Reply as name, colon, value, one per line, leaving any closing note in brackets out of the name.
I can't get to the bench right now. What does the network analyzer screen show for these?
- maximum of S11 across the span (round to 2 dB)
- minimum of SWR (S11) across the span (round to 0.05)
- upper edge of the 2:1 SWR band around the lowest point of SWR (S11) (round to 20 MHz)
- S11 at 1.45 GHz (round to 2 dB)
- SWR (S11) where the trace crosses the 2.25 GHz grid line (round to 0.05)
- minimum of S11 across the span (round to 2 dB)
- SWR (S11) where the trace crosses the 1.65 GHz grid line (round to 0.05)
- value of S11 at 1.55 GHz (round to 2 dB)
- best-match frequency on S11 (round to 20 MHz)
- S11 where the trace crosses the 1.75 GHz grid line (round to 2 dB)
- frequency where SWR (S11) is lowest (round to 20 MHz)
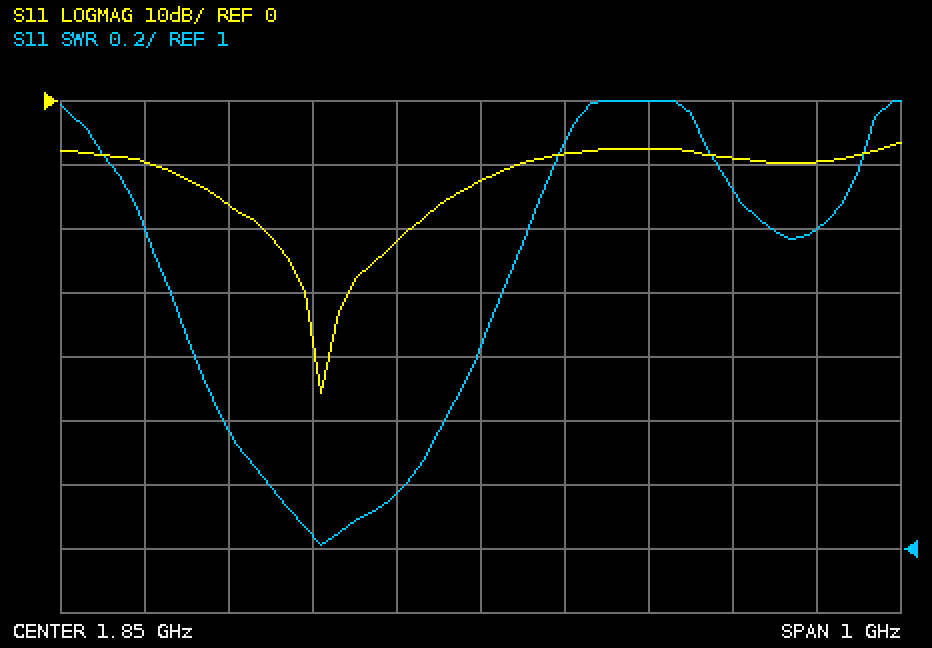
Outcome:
maximum of S11 across the span: -6 dB
minimum of SWR (S11) across the span: 1.00
upper edge of the 2:1 SWR band around the lowest point of SWR (S11): 1.90 GHz
S11 at 1.45 GHz: -10 dB
SWR (S11) where the trace crosses the 2.25 GHz grid line: 2.00
minimum of S11 across the span: -46 dB
SWR (S11) where the trace crosses the 1.65 GHz grid line: 1.05
value of S11 at 1.55 GHz: -16 dB
best-match frequency on S11: 1.66 GHz
S11 where the trace crosses the 1.75 GHz grid line: -22 dB
frequency where SWR (S11) is lowest: 1.66 GHz
